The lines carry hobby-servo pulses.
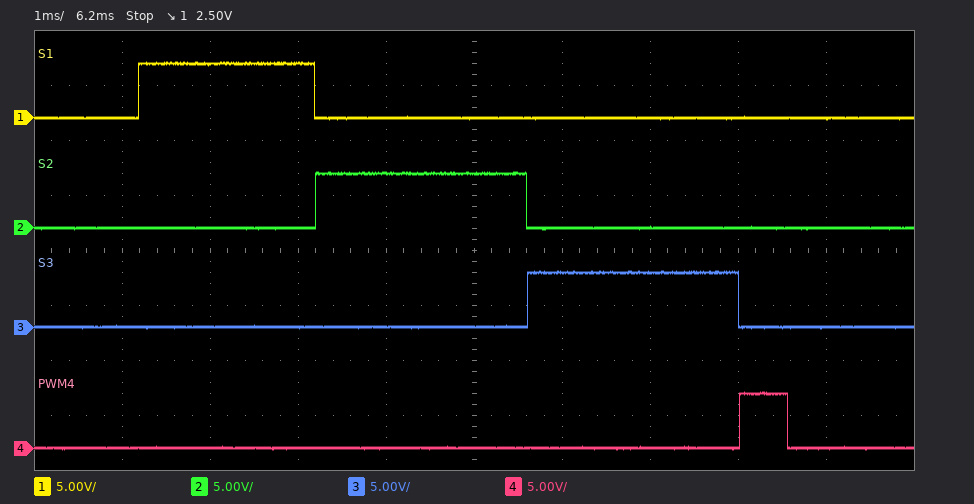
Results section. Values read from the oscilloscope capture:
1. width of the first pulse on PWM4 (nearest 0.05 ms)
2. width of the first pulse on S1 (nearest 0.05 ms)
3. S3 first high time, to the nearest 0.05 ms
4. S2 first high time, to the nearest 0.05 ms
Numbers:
0.55 ms
2.00 ms
2.40 ms
2.40 ms
